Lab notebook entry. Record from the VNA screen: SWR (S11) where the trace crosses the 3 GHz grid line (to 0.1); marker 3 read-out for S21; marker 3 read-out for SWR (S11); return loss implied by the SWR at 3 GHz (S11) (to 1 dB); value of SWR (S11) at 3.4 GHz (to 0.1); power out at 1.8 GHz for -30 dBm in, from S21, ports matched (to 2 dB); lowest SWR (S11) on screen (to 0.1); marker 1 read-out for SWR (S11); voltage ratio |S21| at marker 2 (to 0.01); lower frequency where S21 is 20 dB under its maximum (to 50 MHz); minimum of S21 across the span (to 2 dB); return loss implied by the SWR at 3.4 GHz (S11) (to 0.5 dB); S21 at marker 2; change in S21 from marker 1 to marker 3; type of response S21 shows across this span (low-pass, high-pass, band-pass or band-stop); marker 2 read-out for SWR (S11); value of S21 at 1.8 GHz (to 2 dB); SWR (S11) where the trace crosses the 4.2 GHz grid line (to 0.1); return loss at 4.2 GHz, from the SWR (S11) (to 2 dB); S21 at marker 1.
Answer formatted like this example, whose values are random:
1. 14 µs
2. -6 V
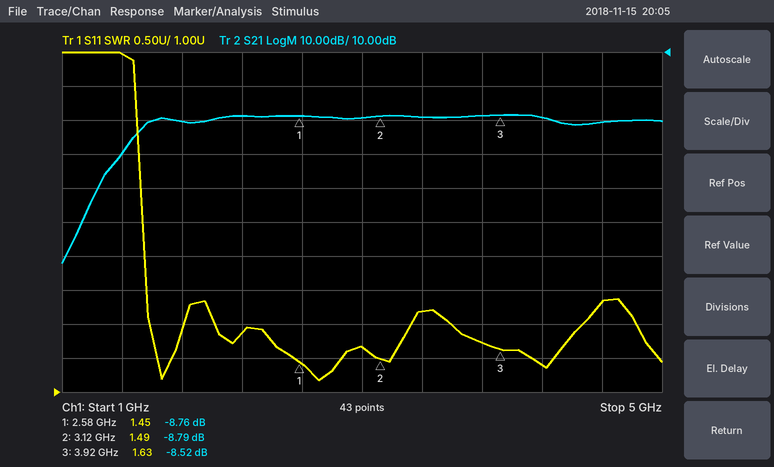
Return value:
1. 1.7
2. -8.52 dB
3. 1.63
4. 12 dB
5. 2.2
6. -40 dBm
7. 1.2
8. 1.45
9. 0.36
10. 1.25 GHz
11. -52 dB
12. 8.5 dB
13. -8.79 dB
14. 0.24 dB
15. high-pass
16. 1.49
17. -10 dB
18. 1.4
19. 16 dB
20. -8.76 dB
